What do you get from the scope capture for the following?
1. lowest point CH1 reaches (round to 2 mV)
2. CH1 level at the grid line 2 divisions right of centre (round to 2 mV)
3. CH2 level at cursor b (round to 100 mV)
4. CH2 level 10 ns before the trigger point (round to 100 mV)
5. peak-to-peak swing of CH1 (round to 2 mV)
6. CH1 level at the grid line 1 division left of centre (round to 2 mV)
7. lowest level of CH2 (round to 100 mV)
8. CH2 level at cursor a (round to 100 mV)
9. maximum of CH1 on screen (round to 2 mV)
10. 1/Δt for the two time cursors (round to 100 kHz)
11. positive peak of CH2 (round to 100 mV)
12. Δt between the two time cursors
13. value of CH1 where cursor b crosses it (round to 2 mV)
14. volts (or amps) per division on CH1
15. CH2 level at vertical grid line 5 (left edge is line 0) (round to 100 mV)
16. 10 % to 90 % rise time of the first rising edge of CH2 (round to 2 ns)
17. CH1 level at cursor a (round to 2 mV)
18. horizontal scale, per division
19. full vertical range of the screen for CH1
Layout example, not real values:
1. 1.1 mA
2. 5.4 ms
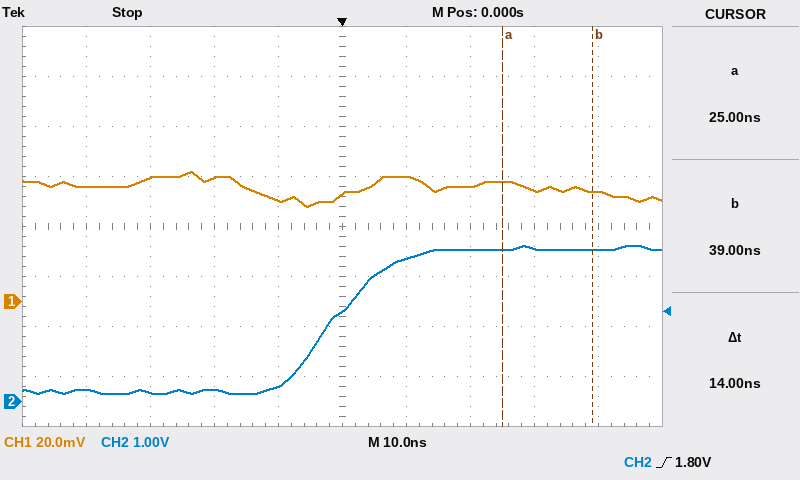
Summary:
1. 38 mV
2. 46 mV
3. 3.0 V
4. 300 mV
5. 14 mV
6. 40 mV
7. 200 mV
8. 3.0 V
9. 52 mV
10. 71.4 MHz
11. 3.1 V
12. 14 ns
13. 44 mV
14. 20 mV
15. 1.8 V
16. 16 ns
17. 48 mV
18. 10 ns
19. 160 mV
